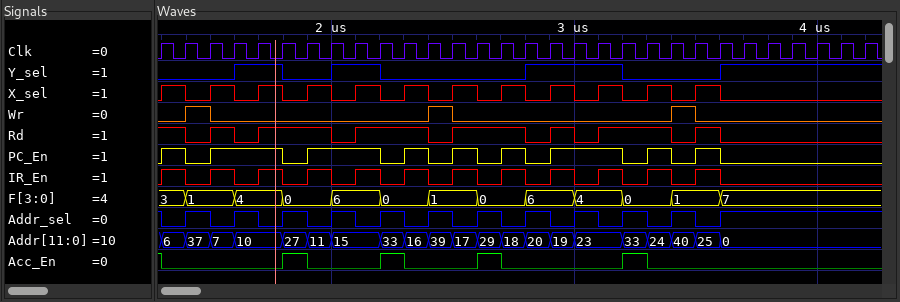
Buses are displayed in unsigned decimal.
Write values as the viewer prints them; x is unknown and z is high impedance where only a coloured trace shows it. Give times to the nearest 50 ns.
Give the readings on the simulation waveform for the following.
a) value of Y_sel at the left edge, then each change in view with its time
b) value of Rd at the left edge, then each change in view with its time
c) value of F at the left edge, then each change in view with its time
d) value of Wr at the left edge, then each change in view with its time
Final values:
0, 1 at 1600 ns, 0 at 1800 ns, 1 at 2000 ns, 0 at 2200 ns, 1 at 2800 ns, 0 at 3200 ns, 1 at 3600 ns
1, 0 at 1400 ns, 1 at 1500 ns, 0 at 1600 ns, 1 at 1700 ns, 0 at 2000 ns, 1 at 2100 ns, 0 at 2400 ns, 1 at 2500 ns, 0 at 2800 ns, 1 at 2900 ns, 0 at 3000 ns, 1 at 3100 ns, 0 at 3400 ns, 1 at 3500 ns, 0 at 3600 ns
3, 1 at 1400 ns, 4 at 1600 ns, 0 at 1800 ns, 6 at 2000 ns, 0 at 2200 ns, 1 at 2400 ns, 0 at 2600 ns, 6 at 2800 ns, 4 at 3000 ns, 0 at 3200 ns, 1 at 3400 ns, 7 at 3600 ns
0, 1 at 1400 ns, 0 at 1500 ns, 1 at 2400 ns, 0 at 2500 ns, 1 at 3400 ns, 0 at 3500 ns
